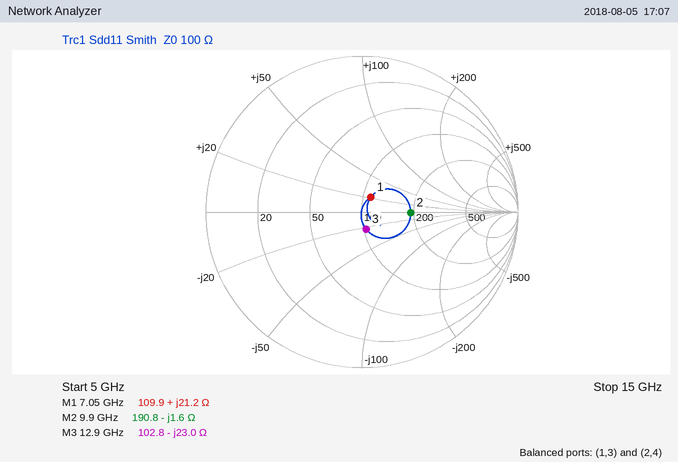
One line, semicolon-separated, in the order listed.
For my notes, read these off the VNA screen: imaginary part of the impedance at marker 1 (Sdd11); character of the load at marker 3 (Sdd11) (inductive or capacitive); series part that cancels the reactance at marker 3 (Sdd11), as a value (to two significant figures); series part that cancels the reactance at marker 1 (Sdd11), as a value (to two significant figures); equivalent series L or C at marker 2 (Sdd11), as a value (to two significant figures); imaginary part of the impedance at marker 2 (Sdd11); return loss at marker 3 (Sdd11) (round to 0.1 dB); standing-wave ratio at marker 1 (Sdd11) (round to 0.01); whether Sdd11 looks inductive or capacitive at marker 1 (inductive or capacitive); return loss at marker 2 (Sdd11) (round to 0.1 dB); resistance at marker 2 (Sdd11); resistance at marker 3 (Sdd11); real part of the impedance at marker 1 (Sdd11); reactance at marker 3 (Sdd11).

+21.2 Ω; capacitive; 280 pH; 1.1 pF; 10 pF; -1.6 Ω; 18.9 dB; 1.25; inductive; 10.1 dB; 190.8 Ω; 102.8 Ω; 109.9 Ω; -23.0 Ω
